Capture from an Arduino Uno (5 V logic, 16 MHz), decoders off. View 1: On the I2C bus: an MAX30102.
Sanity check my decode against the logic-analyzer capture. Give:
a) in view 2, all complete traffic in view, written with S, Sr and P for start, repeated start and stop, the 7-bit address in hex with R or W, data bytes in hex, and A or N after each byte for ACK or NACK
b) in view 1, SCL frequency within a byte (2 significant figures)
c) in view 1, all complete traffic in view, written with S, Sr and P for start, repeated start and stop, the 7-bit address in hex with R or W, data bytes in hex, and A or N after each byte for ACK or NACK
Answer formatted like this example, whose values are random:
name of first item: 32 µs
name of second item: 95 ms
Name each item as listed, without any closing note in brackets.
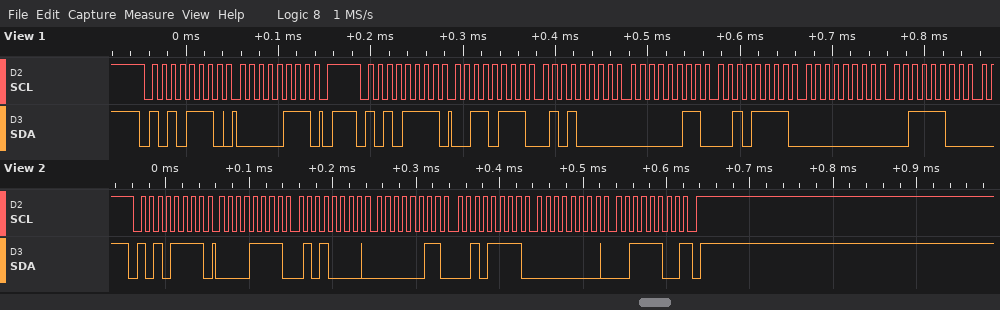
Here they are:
in view 2, all complete traffic in view, written with S, Sr and P for start, repeated start and stop, the 7-bit address in hex with R or W, data bytes in hex, and A or N after each byte for ACK or NACK: S 57R A 0F A 50 A 03 A 2F A 00 A 3C N P
in view 1, SCL frequency within a byte: 100 kHz
in view 1, all complete traffic in view, written with S, Sr and P for start, repeated start and stop, the 7-bit address in hex with R or W, data bytes in hex, and A or N after each byte for ACK or NACK: S 57W A 07 A P S 57R A 37 A 50 A 03 A 2F A 00 A 3C A
